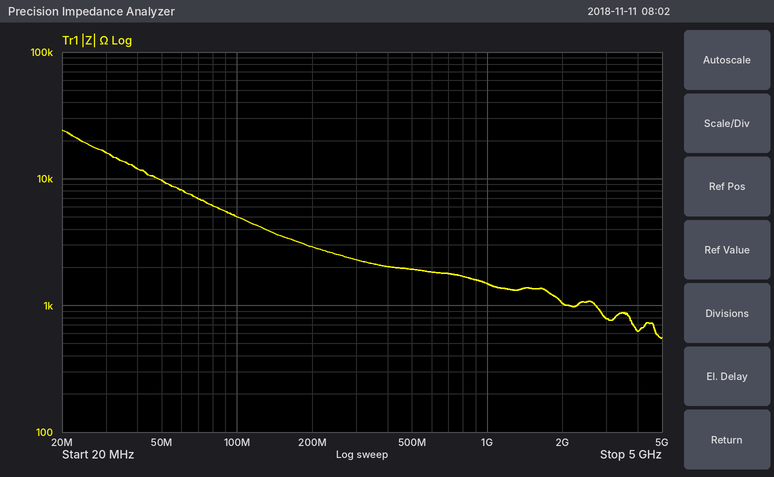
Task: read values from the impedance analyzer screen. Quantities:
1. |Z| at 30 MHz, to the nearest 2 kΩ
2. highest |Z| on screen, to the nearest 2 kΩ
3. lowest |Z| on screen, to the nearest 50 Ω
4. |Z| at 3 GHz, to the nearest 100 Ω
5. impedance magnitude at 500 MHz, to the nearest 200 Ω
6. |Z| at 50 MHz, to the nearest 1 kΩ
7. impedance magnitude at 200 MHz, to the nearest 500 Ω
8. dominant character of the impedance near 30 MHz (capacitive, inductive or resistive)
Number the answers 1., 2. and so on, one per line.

1. 16 kΩ
2. 24 kΩ
3. 550 Ω
4. 800 Ω
5. 2.0 kΩ
6. 10 kΩ
7. 3.0 kΩ
8. capacitive
